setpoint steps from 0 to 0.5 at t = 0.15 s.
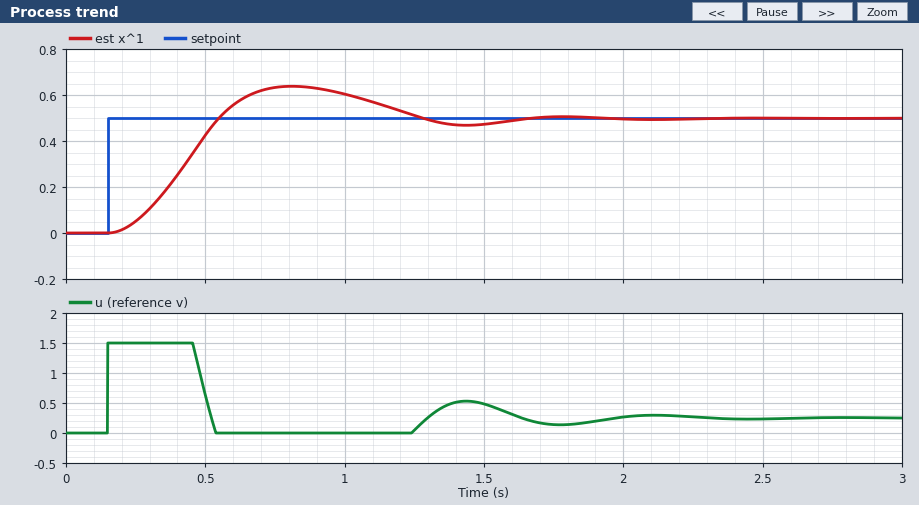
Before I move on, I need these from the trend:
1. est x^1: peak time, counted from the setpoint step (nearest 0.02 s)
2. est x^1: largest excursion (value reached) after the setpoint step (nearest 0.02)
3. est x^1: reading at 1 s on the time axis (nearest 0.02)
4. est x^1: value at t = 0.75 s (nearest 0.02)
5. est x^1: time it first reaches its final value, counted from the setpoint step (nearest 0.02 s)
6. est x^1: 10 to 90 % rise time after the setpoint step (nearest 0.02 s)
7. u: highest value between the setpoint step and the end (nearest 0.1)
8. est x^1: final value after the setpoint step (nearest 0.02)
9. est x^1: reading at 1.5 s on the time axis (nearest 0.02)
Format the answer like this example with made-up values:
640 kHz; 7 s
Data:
0.66 s; 0.64; 0.60; 0.64; 0.40 s; 0.26 s; 1.5; 0.50; 0.48
